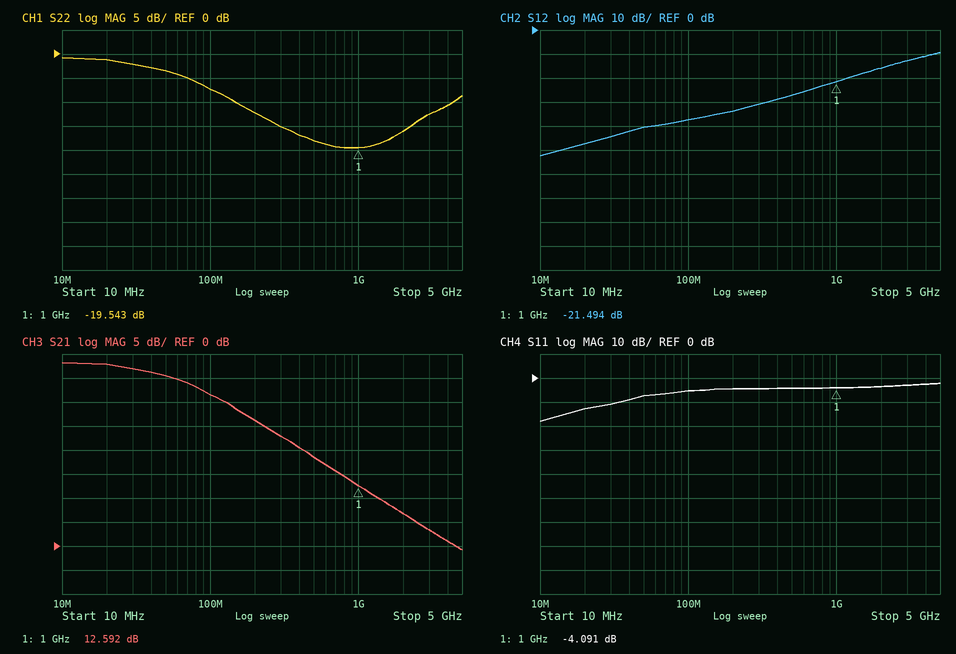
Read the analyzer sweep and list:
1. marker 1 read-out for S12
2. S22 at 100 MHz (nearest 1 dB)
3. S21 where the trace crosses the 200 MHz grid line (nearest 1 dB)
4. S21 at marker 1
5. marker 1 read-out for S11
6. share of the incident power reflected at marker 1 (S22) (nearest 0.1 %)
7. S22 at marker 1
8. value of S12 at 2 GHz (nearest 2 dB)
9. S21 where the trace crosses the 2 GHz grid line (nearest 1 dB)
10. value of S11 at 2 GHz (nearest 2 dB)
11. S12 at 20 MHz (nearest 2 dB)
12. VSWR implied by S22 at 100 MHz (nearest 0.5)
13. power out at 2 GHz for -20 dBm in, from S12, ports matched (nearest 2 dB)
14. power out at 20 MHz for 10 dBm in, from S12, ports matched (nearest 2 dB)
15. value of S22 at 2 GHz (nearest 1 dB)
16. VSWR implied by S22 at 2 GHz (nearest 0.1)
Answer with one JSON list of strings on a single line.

["-21.494 dB", "-7 dB", "26 dB", "12.592 dB", "-4.091 dB", "1.1 %", "-19.543 dB", "-16 dB", "7 dB", "-4 dB", "-48 dB", "2.5", "-36 dBm", "-38 dBm", "-16 dB", "1.4"]
